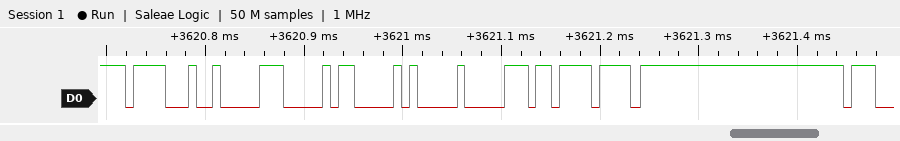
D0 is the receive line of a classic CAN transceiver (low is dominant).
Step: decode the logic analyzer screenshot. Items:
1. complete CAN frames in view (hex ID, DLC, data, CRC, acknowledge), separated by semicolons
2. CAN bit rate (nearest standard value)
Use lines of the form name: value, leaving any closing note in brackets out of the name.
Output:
complete CAN frames in view (hex ID, DLC, data, CRC, acknowledge), separated by semicolons: ID 789, DLC 3, data 03 02 00, CRC 36F7, ACK
CAN bit rate: 125 kbit/s
